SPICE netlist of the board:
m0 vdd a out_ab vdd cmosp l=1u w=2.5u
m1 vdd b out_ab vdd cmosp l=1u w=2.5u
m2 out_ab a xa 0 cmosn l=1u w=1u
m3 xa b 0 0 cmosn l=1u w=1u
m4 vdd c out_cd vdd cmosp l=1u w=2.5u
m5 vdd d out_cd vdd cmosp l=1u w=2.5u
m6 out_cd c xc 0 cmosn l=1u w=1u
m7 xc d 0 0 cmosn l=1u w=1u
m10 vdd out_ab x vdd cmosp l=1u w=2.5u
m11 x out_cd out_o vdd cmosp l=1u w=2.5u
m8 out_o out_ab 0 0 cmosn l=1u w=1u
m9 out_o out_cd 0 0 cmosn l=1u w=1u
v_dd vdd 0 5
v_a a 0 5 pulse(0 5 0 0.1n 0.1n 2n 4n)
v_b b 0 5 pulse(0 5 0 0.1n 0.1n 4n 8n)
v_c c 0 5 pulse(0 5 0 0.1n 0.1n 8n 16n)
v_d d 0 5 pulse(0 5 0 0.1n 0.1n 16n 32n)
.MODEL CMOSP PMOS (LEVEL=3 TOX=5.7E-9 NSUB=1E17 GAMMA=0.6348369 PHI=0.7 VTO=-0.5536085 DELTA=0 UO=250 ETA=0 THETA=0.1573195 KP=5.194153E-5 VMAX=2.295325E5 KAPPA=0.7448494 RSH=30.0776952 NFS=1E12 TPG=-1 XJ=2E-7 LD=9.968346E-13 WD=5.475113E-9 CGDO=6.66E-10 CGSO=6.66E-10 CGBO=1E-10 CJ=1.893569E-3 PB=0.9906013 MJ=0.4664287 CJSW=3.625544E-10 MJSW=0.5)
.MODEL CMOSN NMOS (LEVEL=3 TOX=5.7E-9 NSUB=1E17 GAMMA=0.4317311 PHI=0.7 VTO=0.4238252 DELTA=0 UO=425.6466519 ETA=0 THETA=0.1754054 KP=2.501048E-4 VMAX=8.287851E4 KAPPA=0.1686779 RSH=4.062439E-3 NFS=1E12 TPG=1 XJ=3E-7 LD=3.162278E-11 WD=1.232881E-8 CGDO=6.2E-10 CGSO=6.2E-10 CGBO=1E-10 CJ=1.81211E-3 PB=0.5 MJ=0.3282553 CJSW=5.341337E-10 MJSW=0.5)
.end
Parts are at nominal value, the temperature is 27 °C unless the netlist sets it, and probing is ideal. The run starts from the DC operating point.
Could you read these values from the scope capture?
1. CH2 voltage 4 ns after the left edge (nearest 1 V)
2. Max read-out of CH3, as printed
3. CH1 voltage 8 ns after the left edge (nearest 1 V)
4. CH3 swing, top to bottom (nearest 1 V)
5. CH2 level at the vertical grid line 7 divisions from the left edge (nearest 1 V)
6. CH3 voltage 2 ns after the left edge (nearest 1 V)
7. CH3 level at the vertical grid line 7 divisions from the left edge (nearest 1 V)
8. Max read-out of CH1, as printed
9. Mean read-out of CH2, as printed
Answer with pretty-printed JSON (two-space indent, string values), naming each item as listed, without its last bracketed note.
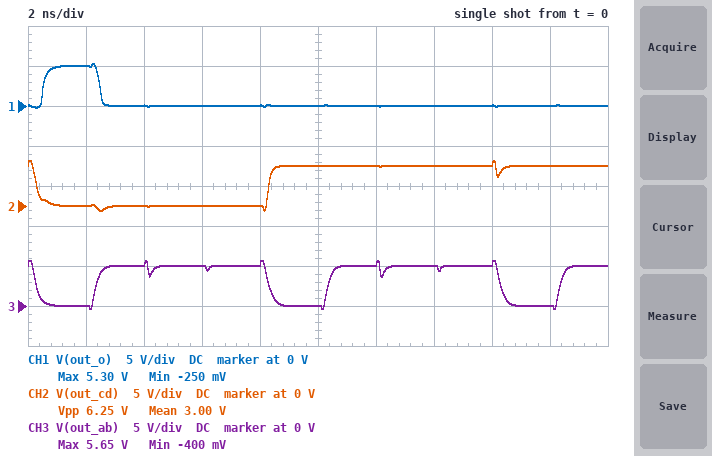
{
  "CH2 voltage 4 ns after the left edge": "0 V",
  "Max read-out of CH3, as printed": "5.65 V",
  "CH1 voltage 8 ns after the left edge": "0 V",
  "CH3 swing, top to bottom": "6 V",
  "CH2 level at the vertical grid line 7 divisions from the left edge": "5 V",
  "CH3 voltage 2 ns after the left edge": "0 V",
  "CH3 level at the vertical grid line 7 divisions from the left edge": "5 V",
  "Max read-out of CH1, as printed": "5.30 V",
  "Mean read-out of CH2, as printed": "3.00 V"
}
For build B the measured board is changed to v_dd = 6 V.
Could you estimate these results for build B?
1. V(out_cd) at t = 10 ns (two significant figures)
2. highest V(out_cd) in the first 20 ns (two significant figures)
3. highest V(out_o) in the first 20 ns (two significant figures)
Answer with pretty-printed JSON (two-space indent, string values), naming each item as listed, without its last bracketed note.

{
  "V(out_cd) at t = 10 ns": "6.0 V",
  "highest V(out_cd) in the first 20 ns": "6.6 V",
  "highest V(out_o) in the first 20 ns": "6.3 V"
}
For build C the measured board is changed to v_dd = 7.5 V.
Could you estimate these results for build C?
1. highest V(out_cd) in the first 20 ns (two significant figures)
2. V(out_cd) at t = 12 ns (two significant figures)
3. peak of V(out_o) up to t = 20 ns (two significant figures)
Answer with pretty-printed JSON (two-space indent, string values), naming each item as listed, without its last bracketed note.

{
  "highest V(out_cd) in the first 20 ns": "8.1 V",
  "V(out_cd) at t = 12 ns": "7.5 V",
  "peak of V(out_o) up to t = 20 ns": "6.5 V"
}
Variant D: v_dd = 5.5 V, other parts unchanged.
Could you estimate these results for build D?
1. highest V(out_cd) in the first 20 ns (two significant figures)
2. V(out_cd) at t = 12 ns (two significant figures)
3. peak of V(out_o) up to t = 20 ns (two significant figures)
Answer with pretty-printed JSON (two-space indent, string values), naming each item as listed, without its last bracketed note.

{
  "highest V(out_cd) in the first 20 ns": "6.1 V",
  "V(out_cd) at t = 12 ns": "5.5 V",
  "peak of V(out_o) up to t = 20 ns": "5.8 V"
}
